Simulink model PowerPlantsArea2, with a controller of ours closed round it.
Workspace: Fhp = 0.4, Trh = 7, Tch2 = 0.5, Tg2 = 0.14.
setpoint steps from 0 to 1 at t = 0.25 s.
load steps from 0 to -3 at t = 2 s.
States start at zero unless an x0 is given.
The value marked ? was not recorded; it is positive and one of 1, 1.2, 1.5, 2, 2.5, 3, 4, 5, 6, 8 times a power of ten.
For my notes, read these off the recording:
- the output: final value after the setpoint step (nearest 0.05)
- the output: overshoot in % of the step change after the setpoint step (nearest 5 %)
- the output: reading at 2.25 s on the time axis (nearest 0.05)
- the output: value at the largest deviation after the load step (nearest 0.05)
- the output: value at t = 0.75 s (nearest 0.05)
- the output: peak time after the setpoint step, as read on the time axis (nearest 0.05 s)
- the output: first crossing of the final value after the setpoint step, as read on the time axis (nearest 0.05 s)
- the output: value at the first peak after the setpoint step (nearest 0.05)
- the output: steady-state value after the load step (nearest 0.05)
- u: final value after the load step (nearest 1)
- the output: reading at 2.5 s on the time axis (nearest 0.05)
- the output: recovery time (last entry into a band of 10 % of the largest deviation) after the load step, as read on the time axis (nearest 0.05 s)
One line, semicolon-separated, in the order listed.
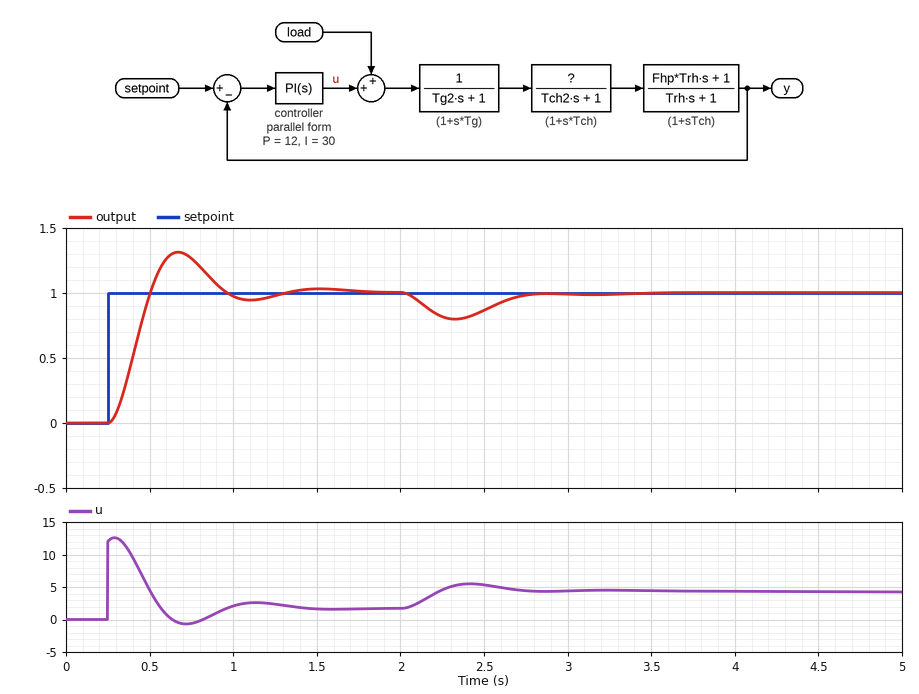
1.00; 30 %; 0.80; 0.80; 1.25; 0.65 s; 0.50 s; 1.30; 1.00; 4; 0.85; 2.75 s
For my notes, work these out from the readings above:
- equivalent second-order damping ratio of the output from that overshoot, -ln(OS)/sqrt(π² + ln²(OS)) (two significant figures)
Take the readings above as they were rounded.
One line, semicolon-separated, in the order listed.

0.36
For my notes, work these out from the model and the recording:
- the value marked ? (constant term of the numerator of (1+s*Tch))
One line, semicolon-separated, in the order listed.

1
